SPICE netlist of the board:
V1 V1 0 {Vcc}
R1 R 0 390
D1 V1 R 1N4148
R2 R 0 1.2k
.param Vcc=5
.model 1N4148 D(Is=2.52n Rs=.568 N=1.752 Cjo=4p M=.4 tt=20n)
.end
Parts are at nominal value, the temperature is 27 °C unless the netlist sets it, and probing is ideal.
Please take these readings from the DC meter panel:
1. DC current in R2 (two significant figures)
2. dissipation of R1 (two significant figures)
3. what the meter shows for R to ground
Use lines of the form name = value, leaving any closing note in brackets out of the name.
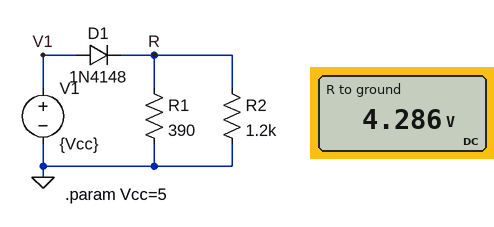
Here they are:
DC current in R2 = 3.6 mA
dissipation of R1 = 47 mW
what the meter shows for R to ground = 4.286 V
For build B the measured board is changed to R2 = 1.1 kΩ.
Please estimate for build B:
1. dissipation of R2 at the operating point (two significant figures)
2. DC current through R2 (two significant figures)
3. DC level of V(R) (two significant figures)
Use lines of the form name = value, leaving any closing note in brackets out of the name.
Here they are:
dissipation of R2 at the operating point = 17 mW
DC current through R2 = 3.9 mA
DC level of V(R) = 4.3 V
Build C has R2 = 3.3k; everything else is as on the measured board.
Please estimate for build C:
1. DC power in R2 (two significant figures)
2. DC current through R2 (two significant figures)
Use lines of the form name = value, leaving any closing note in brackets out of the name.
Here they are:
DC power in R2 = 5.6 mW
DC current through R2 = 1.3 mA
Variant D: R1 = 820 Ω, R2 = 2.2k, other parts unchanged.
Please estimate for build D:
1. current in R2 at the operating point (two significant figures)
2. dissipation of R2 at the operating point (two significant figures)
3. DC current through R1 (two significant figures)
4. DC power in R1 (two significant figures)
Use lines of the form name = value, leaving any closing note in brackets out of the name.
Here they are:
current in R2 at the operating point = 2.0 mA
dissipation of R2 at the operating point = 8.5 mW
DC current through R1 = 5.3 mA
DC power in R1 = 23 mW
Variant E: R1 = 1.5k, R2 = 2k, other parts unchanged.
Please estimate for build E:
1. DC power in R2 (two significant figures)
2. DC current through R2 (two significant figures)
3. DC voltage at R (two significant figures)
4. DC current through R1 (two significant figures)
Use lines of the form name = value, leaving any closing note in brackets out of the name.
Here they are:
DC power in R2 = 9.4 mW
DC current through R2 = 2.2 mA
DC voltage at R = 4.3 V
DC current through R1 = 2.9 mA
